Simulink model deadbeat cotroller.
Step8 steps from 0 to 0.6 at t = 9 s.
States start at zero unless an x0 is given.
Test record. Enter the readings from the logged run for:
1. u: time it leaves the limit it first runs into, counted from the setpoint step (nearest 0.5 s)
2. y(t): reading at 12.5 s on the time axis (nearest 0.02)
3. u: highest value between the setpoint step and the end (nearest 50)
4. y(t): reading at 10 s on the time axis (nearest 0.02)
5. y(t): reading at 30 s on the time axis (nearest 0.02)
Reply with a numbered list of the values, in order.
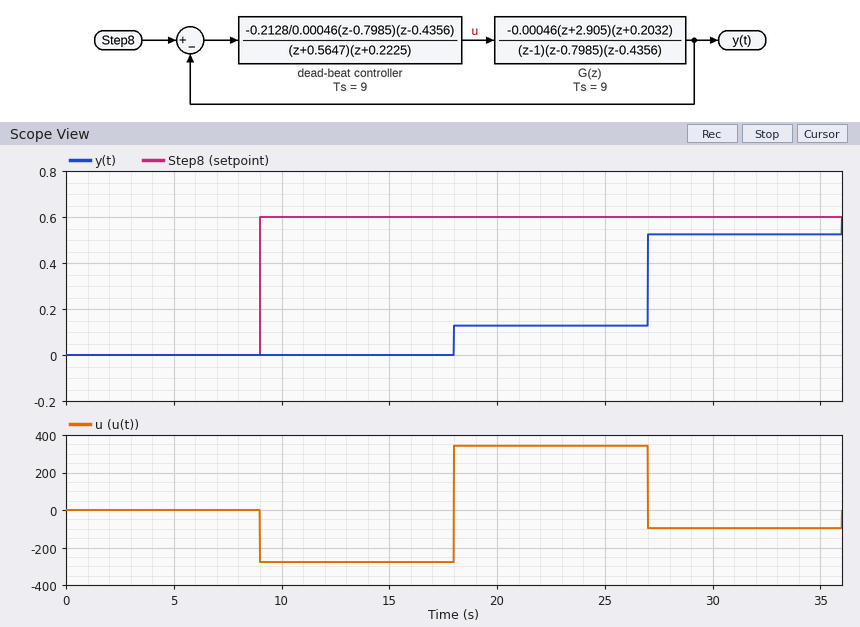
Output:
1. 9.0 s
2. 0.00
3. 350
4. 0.00
5. 0.52
